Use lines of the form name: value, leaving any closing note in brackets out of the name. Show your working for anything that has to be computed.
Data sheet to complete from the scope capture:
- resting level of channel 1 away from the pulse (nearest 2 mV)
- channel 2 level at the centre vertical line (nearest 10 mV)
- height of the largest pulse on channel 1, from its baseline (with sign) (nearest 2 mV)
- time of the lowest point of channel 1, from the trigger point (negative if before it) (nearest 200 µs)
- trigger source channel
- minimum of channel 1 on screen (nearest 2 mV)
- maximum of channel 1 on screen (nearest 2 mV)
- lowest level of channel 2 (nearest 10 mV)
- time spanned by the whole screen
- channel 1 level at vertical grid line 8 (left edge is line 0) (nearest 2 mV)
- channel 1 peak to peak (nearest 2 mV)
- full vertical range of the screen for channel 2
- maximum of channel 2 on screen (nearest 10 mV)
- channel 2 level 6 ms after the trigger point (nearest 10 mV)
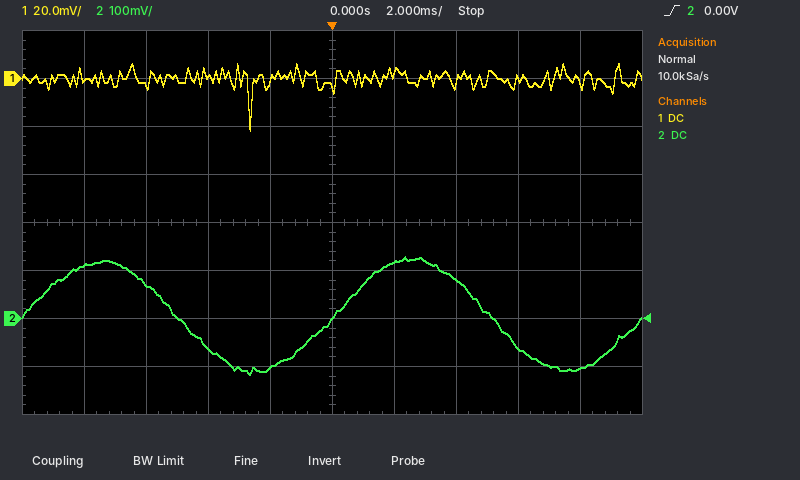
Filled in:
resting level of channel 1 away from the pulse: 0 mV
channel 2 level at the centre vertical line: 0 mV
height of the largest pulse on channel 1, from its baseline (with sign): -22 mV − (0 mV) = -22 mV
time of the lowest point of channel 1, from the trigger point (negative if before it): -2.6 ms
trigger source channel: channel 2
minimum of channel 1 on screen: -22 mV
maximum of channel 1 on screen: 6 mV
lowest level of channel 2: -120 mV
time spanned by the whole screen: 20 ms
channel 1 level at vertical grid line 8 (left edge is line 0): 0 mV
channel 1 peak to peak: 6 mV − (-22 mV) = 28 mV
full vertical range of the screen for channel 2: 800 mV
maximum of channel 2 on screen: 130 mV
channel 2 level 6 ms after the trigger point: -60 mV
